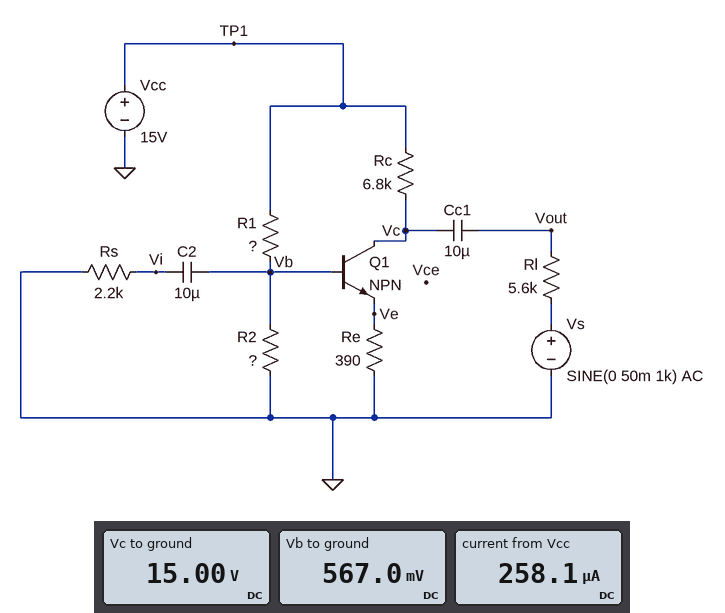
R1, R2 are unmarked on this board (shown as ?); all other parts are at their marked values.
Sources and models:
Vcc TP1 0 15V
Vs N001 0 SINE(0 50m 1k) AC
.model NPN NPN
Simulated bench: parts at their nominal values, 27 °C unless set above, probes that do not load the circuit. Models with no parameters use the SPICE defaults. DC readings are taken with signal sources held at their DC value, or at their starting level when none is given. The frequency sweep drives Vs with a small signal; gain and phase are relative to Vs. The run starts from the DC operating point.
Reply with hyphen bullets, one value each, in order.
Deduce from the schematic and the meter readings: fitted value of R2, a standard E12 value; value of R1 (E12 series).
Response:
- 2.2 kΩ
- 56 kΩ
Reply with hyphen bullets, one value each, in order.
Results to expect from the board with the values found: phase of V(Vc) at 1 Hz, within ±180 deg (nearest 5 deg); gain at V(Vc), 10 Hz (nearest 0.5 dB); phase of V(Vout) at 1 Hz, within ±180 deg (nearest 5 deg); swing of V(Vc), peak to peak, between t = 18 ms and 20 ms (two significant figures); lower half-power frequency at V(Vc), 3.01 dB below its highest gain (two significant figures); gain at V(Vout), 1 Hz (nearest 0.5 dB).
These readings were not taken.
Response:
- 50 deg
- -5.5 dB
- -15 deg
- 55 mV
- 1.3 Hz
- -1.5 dB
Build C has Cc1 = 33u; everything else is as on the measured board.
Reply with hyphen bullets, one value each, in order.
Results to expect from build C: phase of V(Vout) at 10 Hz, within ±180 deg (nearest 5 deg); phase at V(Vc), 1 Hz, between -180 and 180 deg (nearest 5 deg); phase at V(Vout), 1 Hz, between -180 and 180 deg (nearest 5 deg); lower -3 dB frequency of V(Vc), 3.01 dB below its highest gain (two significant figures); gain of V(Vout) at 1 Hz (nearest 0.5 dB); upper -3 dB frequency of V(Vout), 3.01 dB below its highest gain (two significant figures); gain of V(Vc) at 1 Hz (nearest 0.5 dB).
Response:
- 0 deg
- 20 deg
- -15 deg
- 390 mHz
- -4.0 dB
- 620 mHz
- -6.0 dB
